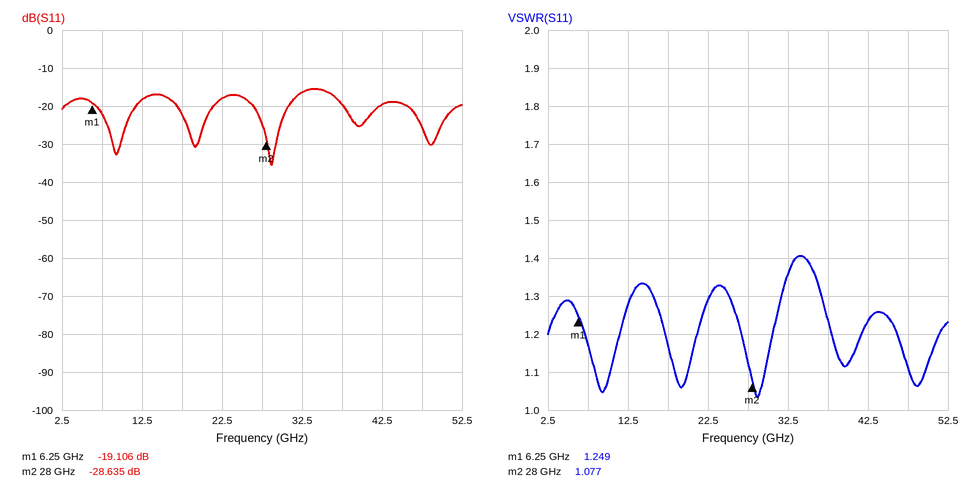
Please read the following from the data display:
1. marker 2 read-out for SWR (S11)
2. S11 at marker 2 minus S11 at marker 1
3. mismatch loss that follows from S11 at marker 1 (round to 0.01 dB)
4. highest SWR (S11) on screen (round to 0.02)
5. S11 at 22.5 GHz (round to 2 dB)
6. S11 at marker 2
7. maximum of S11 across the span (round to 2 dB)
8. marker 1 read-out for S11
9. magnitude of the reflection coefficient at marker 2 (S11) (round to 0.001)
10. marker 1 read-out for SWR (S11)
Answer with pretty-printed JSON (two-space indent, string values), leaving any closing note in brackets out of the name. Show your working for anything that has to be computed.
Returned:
{
  "marker 2 read-out for SWR": "1.077",
  "S11 at marker 2 minus S11 at marker 1": "-28.635 − (-19.106) = -9.529 dB",
  "mismatch loss that follows from S11 at marker 1": "−10 log10(1 − 10^(-19.106/10)) ≈ 0.05 dB",
  "highest SWR (S11) on screen": "1.40",
  "S11 at 22.5 GHz": "-18 dB",
  "S11 at marker 2": "-28.635 dB",
  "maximum of S11 across the span": "-16 dB",
  "marker 1 read-out for S11": "-19.106 dB",
  "magnitude of the reflection coefficient at marker 2 (S11)": "10^(-28.635/20) ≈ 0.037",
  "marker 1 read-out for SWR": "1.249"
}
